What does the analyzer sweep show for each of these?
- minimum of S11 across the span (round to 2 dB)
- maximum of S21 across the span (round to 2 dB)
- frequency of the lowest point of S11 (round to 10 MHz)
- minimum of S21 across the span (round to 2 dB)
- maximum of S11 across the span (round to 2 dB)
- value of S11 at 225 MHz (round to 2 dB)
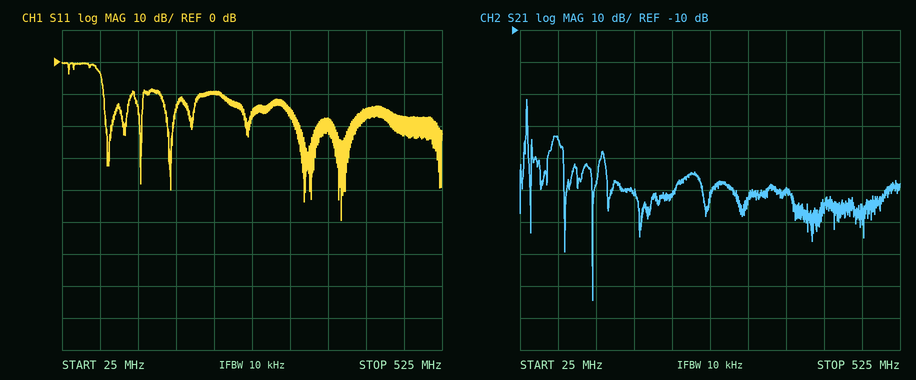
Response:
-50 dB
-32 dB
390 MHz
-94 dB
0 dB
-10 dB
